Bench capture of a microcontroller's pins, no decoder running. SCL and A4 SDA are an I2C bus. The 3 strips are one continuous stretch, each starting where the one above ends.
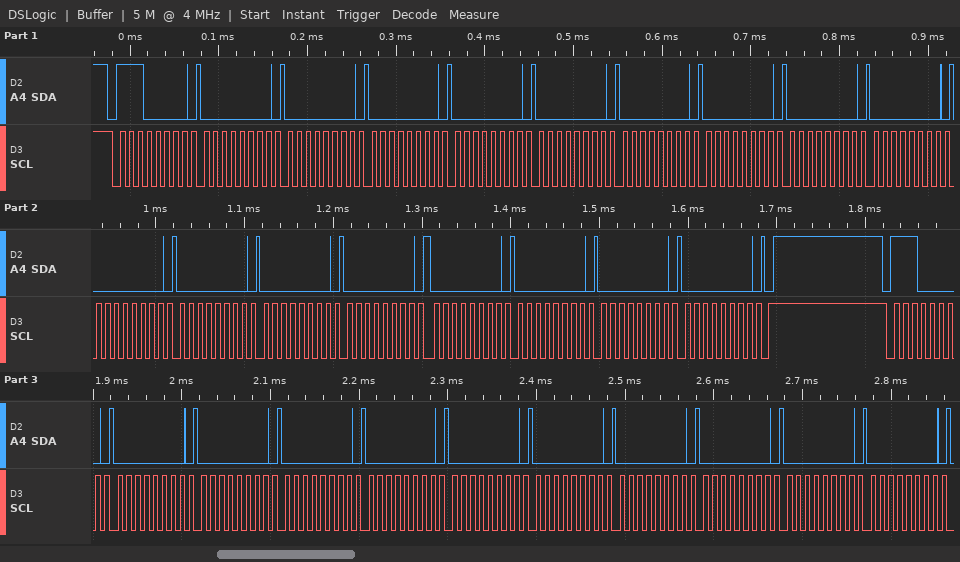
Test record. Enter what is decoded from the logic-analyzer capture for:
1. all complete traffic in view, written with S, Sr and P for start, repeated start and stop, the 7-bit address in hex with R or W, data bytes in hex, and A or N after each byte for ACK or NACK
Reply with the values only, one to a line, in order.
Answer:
S 70W A 00 A 00 A 00 A 00 A 00 A 00 A 00 A 00 A 00 A 00 A 00 A 00 A 00 A 00 A 00 A 00 A 00 A P S 70W A 00 A 00 A 00 A 00 A 00 A 00 A 00 A 00 A 00 A 00 A
